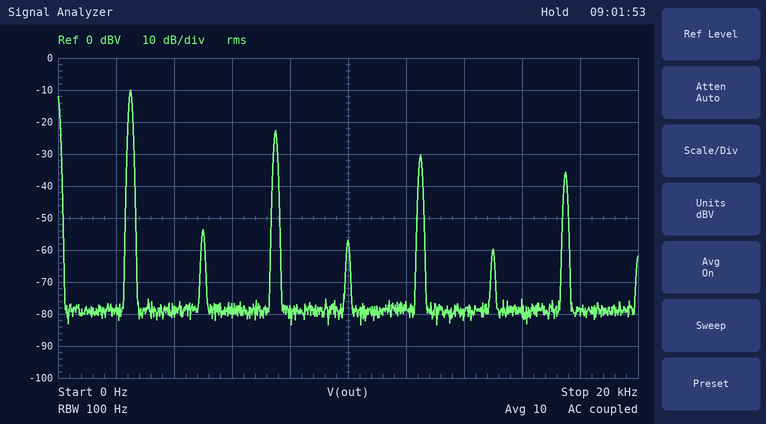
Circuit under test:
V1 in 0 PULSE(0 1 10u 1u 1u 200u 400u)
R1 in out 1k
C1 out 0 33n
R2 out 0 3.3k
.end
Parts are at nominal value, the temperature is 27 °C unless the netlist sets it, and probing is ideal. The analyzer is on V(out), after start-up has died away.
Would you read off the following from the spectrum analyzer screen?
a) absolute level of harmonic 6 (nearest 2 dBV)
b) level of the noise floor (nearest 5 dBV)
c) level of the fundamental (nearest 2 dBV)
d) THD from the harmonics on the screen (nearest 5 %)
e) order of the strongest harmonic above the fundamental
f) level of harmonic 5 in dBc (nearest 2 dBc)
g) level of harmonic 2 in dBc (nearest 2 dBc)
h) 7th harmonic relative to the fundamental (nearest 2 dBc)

-60 dBV
-80 dBV
-10 dBV
25 %
3
-20 dBc
-44 dBc
-26 dBc
